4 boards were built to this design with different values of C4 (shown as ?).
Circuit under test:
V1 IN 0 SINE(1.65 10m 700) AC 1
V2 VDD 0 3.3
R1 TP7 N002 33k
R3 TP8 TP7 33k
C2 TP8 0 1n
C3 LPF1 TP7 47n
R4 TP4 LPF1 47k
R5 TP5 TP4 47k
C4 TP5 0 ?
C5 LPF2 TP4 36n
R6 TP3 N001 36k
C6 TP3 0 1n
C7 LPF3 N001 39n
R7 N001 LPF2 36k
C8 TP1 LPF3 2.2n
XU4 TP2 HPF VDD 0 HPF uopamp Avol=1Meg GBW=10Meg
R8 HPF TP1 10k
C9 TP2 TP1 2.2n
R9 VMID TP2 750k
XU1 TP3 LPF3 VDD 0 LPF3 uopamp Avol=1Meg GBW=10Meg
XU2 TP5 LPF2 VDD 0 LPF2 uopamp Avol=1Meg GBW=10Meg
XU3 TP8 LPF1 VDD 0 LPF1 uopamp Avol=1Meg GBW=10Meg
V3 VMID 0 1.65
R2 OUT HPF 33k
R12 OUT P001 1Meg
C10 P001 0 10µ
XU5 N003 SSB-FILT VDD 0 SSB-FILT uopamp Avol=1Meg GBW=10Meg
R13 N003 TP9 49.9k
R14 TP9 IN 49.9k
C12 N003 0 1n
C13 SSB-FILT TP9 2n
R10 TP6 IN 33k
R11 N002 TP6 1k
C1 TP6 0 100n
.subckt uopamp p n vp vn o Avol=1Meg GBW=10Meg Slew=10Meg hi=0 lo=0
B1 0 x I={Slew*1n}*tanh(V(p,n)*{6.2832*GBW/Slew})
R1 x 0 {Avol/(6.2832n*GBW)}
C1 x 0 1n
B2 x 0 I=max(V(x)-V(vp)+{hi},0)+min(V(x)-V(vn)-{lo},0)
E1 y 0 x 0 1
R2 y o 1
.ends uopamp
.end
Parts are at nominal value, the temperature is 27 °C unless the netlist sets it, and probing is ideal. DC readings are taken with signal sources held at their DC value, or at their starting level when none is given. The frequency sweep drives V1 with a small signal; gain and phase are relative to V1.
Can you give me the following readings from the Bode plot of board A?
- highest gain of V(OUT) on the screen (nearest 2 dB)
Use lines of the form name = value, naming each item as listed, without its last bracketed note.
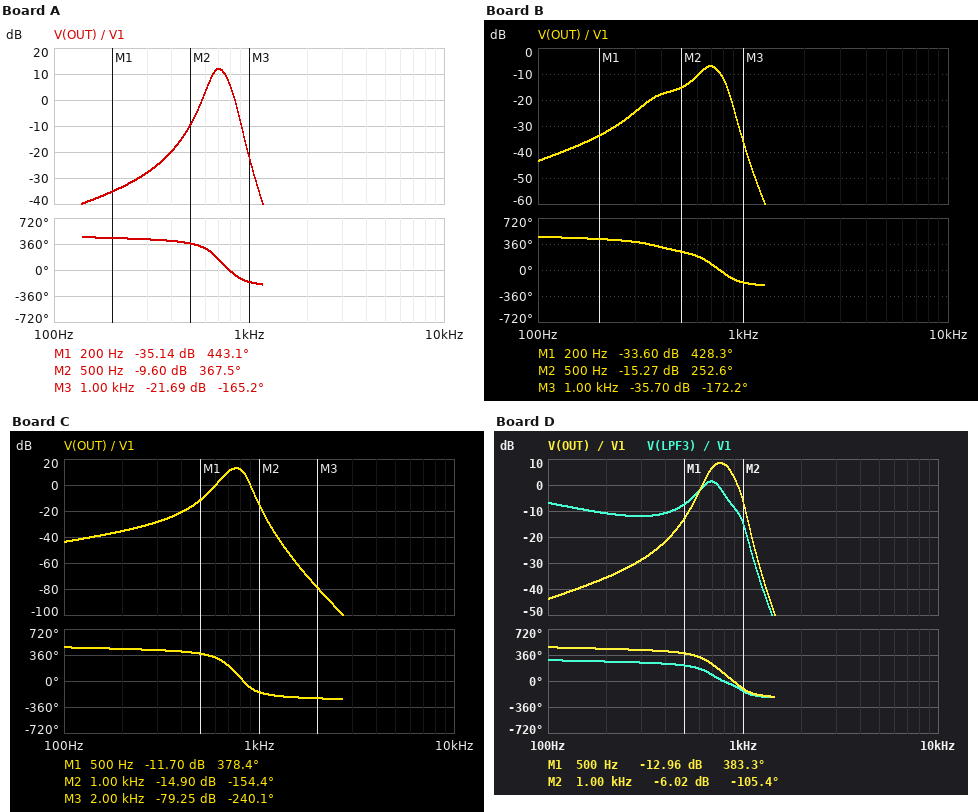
highest gain of V(OUT) on the screen = 12 dB
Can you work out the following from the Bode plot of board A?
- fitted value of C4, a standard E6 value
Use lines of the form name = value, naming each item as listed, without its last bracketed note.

fitted value of C4, a standard E6 value = 680 pF
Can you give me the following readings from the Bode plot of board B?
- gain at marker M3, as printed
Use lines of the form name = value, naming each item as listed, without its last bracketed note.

gain at marker M3, as printed = -35.70 dB
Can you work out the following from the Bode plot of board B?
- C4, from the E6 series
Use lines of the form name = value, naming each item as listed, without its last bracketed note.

C4, from the E6 series = 2.2 nF
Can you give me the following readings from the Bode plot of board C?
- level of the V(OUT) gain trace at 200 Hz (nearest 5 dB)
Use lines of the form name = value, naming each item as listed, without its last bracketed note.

level of the V(OUT) gain trace at 200 Hz = -35 dB
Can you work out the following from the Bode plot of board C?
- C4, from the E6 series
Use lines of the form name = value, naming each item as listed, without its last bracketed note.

C4, from the E6 series = 470 pF
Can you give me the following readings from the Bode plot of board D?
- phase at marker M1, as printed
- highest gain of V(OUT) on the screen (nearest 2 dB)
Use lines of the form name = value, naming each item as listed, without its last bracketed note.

phase at marker M1, as printed = 383.3 deg
highest gain of V(OUT) on the screen = 8 dB
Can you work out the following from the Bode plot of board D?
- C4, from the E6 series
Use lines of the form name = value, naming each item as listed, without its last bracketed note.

C4, from the E6 series = 330 pF
